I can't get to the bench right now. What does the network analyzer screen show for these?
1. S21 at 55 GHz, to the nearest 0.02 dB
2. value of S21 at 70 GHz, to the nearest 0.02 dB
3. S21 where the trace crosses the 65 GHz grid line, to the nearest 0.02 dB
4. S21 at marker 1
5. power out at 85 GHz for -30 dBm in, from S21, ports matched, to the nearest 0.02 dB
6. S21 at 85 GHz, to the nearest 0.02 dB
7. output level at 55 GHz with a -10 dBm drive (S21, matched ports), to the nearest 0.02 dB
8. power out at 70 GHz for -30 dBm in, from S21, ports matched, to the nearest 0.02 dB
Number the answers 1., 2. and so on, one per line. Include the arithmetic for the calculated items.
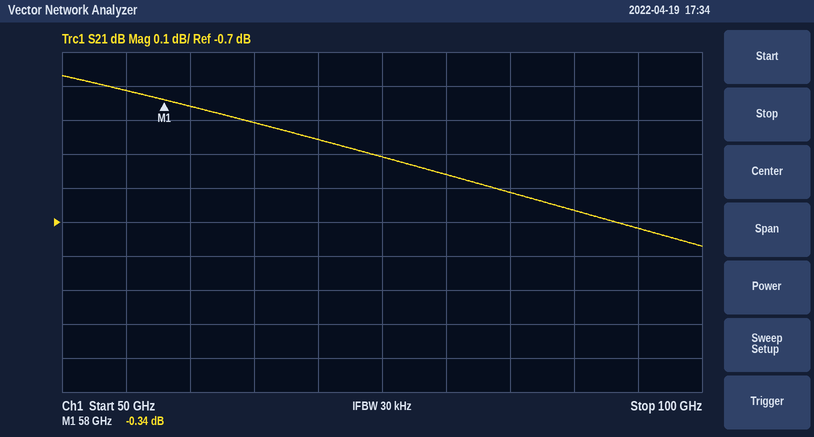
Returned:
1. -0.32 dB
2. -0.46 dB
3. -0.40 dB
4. -0.34 dB
5. -30 dBm + (-0.62 dB) = -30.62 dBm
6. -0.62 dB
7. -10 dBm + (-0.32 dB) = -10.32 dBm
8. -30 dBm + (-0.46 dB) = -30.46 dBm
